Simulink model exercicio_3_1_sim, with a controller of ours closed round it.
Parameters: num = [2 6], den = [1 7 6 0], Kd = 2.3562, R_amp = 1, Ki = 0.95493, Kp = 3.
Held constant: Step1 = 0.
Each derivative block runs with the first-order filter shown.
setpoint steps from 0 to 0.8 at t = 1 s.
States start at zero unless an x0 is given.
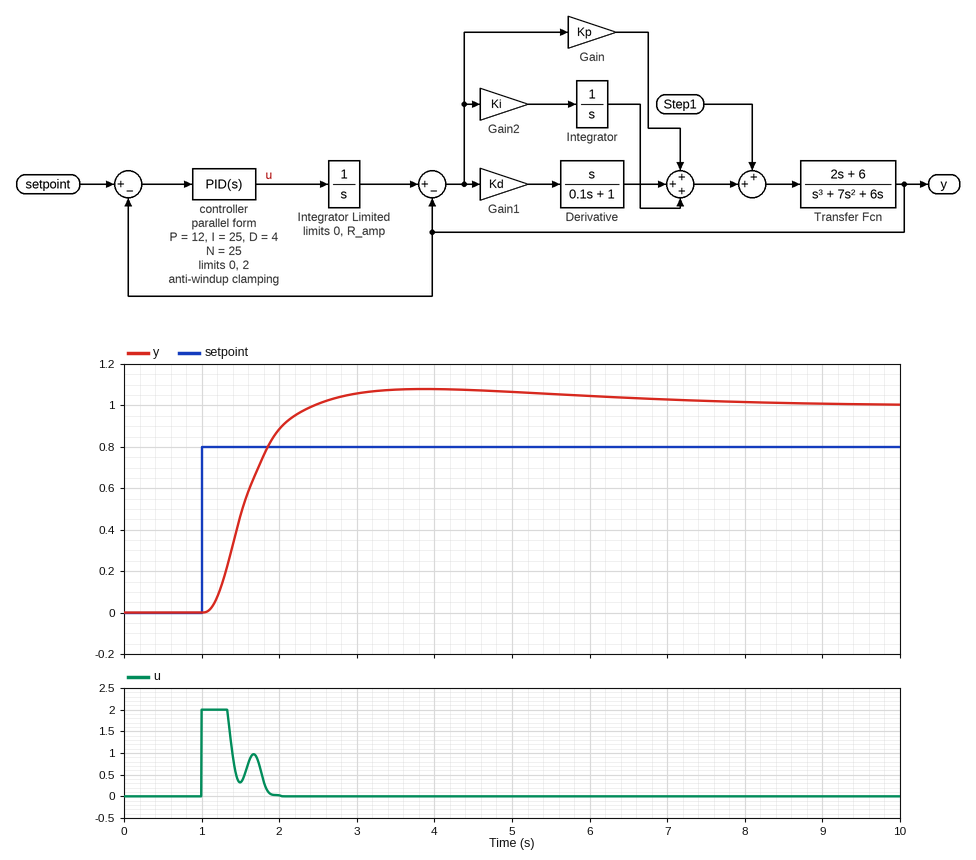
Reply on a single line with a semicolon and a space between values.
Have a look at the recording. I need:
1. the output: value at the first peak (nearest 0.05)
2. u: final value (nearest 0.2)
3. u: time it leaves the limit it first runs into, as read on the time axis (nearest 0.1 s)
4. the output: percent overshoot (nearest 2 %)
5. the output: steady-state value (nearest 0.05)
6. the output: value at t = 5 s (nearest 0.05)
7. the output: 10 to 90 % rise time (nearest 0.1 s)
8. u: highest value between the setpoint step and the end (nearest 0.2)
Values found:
1.10; 0.0; 1.3 s; 8 %; 1.00; 1.05; 0.8 s; 2.0
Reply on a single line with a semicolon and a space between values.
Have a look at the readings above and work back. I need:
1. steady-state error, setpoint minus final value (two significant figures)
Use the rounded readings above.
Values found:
-0.20
